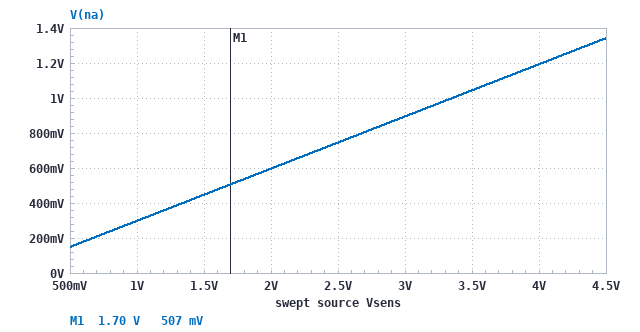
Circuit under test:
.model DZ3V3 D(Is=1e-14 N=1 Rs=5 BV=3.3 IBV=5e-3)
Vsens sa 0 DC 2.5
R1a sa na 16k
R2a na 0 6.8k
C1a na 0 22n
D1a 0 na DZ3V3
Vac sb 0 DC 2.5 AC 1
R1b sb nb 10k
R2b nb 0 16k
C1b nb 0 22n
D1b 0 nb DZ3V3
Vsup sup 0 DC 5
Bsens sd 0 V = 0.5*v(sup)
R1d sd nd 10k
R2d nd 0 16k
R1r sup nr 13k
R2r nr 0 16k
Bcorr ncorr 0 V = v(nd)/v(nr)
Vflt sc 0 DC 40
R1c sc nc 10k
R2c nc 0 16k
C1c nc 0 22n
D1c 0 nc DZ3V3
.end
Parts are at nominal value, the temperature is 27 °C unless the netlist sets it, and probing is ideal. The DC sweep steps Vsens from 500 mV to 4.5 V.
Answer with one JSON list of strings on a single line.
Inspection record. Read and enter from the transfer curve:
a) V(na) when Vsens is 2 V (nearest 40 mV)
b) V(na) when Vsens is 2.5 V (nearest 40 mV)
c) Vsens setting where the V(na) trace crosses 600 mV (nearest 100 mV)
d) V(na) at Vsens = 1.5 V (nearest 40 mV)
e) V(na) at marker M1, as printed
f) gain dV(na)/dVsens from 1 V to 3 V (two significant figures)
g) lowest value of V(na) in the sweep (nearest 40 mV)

["600 mV", "760 mV", "2.0 V", "440 mV", "507 mV", "0.30 V/V", "160 mV"]
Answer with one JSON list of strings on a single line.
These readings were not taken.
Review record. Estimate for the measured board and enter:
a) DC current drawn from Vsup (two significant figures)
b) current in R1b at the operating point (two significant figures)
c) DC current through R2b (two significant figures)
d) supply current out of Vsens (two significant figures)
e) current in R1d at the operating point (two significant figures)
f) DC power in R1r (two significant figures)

["170 µA", "96 µA", "96 µA", "110 µA", "96 µA", "390 µW"]
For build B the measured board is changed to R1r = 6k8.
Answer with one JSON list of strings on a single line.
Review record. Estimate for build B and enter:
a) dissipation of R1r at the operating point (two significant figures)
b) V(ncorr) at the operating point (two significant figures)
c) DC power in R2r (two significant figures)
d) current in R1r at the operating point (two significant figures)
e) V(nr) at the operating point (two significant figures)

["330 µW", "440 mV", "770 µW", "220 µA", "3.5 V"]
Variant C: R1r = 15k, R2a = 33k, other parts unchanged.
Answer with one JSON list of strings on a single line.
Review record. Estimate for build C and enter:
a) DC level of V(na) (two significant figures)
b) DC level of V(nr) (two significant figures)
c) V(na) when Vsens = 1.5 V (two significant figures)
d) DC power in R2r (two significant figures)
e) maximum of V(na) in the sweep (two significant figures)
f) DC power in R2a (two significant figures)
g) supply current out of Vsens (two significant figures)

["1.7 V", "2.6 V", "1.0 V", "420 µW", "3.0 V", "86 µW", "51 µA"]
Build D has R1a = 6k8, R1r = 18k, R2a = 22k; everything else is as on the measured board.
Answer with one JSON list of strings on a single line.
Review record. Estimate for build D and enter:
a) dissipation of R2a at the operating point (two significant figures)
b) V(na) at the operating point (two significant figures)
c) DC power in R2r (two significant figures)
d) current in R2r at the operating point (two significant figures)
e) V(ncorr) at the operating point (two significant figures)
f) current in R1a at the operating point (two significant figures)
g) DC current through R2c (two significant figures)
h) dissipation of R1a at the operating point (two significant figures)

["170 µW", "1.9 V", "350 µW", "150 µA", "650 mV", "87 µA", "210 µA", "51 µW"]
